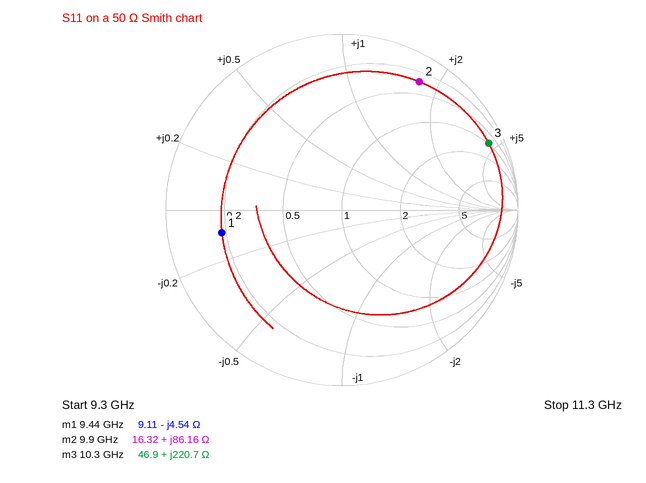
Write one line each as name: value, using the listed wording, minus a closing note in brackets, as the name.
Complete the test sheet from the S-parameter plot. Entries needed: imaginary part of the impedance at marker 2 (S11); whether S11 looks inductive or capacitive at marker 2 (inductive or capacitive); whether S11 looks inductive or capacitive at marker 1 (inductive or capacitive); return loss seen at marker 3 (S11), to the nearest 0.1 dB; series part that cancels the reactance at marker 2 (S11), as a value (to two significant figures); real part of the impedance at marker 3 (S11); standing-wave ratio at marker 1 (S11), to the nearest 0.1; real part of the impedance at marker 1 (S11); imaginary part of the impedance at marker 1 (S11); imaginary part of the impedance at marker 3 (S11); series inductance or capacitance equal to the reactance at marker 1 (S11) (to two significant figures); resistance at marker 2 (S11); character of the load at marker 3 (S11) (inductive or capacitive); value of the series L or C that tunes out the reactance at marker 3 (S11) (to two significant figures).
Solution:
imaginary part of the impedance at marker 2: +86.16 Ω
whether S11 looks inductive or capacitive at marker 2: inductive
whether S11 looks inductive or capacitive at marker 1: capacitive
return loss seen at marker 3 (S11), to the nearest 0.1 dB: 0.8 dB
series part that cancels the reactance at marker 2 (S11), as a value: 190 fF
real part of the impedance at marker 3: 46.9 Ω
standing-wave ratio at marker 1 (S11), to the nearest 0.1: 5.5
real part of the impedance at marker 1: 9.11 Ω
imaginary part of the impedance at marker 1: -4.54 Ω
imaginary part of the impedance at marker 3: +220.7 Ω
series inductance or capacitance equal to the reactance at marker 1 (S11): 3.7 pF
resistance at marker 2: 16.32 Ω
character of the load at marker 3 (S11): inductive
value of the series L or C that tunes out the reactance at marker 3 (S11): 70 fF
